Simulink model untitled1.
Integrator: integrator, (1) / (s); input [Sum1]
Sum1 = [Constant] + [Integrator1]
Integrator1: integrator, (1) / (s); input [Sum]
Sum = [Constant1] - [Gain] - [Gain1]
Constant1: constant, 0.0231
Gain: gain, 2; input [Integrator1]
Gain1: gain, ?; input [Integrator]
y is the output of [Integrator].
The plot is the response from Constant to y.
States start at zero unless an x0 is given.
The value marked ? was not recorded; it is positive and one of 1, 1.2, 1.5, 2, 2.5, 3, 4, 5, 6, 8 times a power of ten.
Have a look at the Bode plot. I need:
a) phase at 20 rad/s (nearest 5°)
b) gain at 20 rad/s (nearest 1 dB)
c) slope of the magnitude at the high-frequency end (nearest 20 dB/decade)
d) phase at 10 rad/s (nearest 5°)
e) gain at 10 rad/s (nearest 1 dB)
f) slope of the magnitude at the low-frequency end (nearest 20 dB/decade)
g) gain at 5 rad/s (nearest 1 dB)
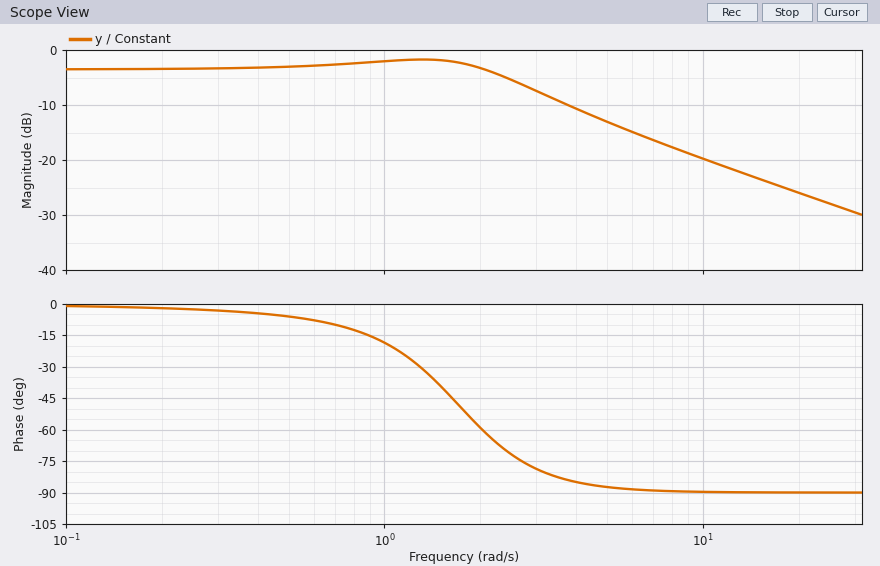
-90°
-26 dB
-20 dB/decade
-90°
-20 dB
0 dB/decade
-13 dB
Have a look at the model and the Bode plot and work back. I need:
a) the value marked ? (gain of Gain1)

3
